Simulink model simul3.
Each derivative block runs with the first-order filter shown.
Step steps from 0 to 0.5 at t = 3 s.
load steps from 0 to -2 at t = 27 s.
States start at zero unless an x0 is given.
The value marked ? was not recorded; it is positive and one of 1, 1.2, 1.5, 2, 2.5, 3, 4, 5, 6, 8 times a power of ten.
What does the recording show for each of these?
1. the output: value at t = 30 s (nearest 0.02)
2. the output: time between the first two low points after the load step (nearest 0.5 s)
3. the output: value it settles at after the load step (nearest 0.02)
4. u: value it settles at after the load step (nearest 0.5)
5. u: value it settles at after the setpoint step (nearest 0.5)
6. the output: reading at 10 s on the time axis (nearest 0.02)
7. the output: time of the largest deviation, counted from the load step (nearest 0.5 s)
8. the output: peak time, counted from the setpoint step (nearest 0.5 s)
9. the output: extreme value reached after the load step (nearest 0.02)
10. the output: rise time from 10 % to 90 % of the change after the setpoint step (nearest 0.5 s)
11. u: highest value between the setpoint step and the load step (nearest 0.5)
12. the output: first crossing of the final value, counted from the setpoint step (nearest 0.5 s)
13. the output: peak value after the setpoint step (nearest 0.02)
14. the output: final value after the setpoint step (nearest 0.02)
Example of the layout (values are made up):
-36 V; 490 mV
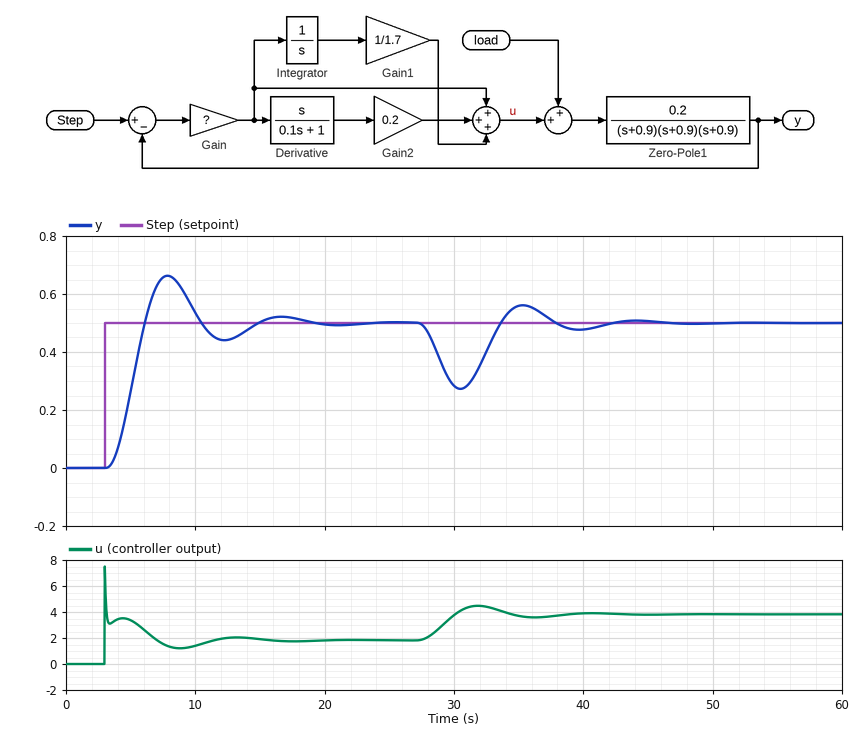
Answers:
0.28; 9.0 s; 0.50; 4.0; 2.0; 0.54; 3.5 s; 5.0 s; 0.28; 2.0 s; 7.5; 3.0 s; 0.66; 0.50
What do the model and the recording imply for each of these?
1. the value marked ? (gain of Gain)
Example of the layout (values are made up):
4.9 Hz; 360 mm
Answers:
5
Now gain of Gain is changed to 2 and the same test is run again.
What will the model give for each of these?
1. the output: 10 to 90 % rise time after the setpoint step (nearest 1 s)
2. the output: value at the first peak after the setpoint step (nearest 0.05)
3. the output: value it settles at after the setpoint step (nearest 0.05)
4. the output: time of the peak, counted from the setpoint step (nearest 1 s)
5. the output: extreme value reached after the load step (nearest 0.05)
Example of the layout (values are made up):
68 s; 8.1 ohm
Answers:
4 s; 0.55; 0.50; 9 s; 0.20
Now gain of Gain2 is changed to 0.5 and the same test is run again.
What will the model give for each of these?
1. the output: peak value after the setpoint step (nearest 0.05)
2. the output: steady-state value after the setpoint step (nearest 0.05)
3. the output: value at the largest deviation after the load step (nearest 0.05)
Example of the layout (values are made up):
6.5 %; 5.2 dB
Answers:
0.60; 0.50; 0.30
